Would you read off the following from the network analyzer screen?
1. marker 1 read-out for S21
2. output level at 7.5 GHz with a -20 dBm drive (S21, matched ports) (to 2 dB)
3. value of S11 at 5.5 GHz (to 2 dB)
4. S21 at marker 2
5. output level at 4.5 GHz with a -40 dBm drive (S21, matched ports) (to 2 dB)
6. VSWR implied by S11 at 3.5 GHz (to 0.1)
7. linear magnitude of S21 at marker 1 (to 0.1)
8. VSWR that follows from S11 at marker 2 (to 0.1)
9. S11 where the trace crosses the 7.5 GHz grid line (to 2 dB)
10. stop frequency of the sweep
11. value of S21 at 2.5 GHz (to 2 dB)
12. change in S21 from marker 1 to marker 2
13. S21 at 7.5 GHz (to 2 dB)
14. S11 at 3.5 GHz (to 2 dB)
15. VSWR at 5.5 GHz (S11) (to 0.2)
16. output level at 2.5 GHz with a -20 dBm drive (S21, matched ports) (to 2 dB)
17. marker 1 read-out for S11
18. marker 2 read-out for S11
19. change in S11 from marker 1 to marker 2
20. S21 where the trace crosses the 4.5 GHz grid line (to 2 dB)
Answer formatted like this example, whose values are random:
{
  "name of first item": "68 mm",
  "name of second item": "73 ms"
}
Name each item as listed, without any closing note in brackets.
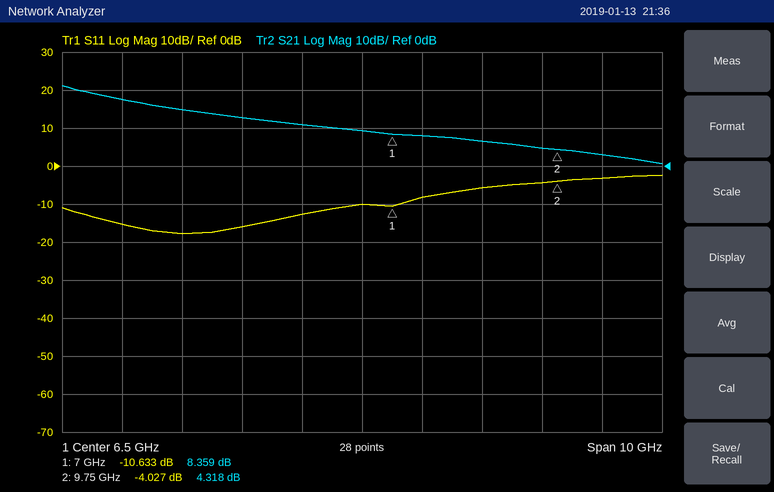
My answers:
{
  "marker 1 read-out for S21": "8.359 dB",
  "output level at 7.5 GHz with a -20 dBm drive (S21, matched ports)": "-12 dBm",
  "value of S11 at 5.5 GHz": "-12 dB",
  "S21 at marker 2": "4.318 dB",
  "output level at 4.5 GHz with a -40 dBm drive (S21, matched ports)": "-28 dBm",
  "VSWR implied by S11 at 3.5 GHz": "1.3",
  "linear magnitude of S21 at marker 1": "2.6",
  "VSWR that follows from S11 at marker 2": "4.4",
  "S11 where the trace crosses the 7.5 GHz grid line": "-8 dB",
  "stop frequency of the sweep": "11.5 GHz",
  "value of S21 at 2.5 GHz": "18 dB",
  "change in S21 from marker 1 to marker 2": "-4.041 dB",
  "S21 at 7.5 GHz": "8 dB",
  "S11 at 3.5 GHz": "-18 dB",
  "VSWR at 5.5 GHz (S11)": "1.6",
  "output level at 2.5 GHz with a -20 dBm drive (S21, matched ports)": "-2 dBm",
  "marker 1 read-out for S11": "-10.633 dB",
  "marker 2 read-out for S11": "-4.027 dB",
  "change in S11 from marker 1 to marker 2": "6.606 dB",
  "S21 where the trace crosses the 4.5 GHz grid line": "12 dB"
}
